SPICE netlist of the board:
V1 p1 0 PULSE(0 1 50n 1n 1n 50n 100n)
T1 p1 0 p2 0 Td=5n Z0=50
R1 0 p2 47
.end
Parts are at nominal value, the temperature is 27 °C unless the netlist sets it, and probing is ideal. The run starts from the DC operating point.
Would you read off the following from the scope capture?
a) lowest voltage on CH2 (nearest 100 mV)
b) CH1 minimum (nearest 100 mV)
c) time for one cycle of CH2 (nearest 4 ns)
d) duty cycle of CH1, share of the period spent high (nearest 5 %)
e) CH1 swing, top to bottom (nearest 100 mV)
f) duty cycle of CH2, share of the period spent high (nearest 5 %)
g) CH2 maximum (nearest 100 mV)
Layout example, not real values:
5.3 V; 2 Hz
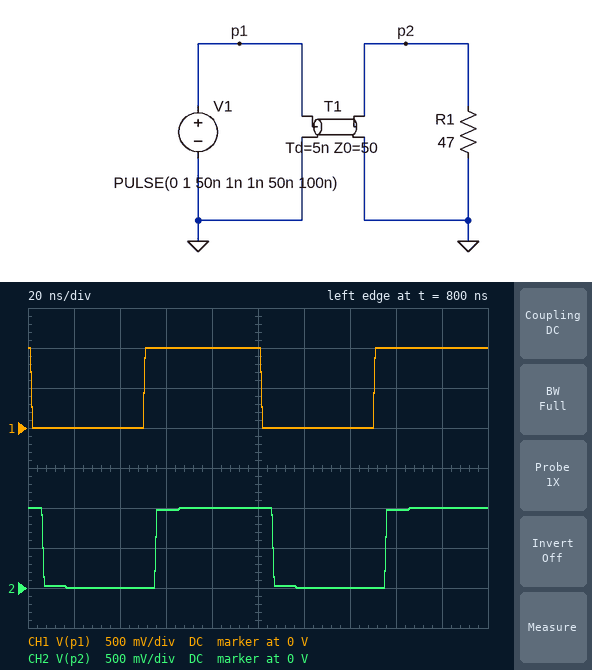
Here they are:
0 V; 0 V; 100 ns; 50 %; 1.0 V; 50 %; 1.0 V
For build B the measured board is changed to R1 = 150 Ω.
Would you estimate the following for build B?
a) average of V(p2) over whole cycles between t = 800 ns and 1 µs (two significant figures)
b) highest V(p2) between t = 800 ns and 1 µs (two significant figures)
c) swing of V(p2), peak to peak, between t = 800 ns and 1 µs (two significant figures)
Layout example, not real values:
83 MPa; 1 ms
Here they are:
510 mV; 1.5 V; 2.0 V
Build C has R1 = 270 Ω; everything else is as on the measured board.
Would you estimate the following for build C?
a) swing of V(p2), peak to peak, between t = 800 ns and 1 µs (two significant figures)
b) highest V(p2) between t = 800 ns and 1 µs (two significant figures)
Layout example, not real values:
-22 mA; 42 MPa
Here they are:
2.6 V; 1.8 V
